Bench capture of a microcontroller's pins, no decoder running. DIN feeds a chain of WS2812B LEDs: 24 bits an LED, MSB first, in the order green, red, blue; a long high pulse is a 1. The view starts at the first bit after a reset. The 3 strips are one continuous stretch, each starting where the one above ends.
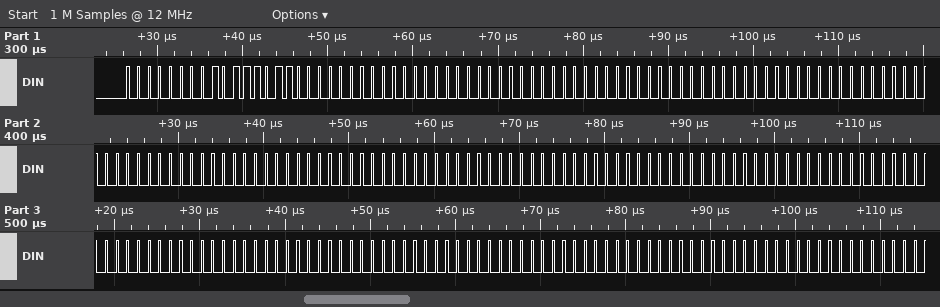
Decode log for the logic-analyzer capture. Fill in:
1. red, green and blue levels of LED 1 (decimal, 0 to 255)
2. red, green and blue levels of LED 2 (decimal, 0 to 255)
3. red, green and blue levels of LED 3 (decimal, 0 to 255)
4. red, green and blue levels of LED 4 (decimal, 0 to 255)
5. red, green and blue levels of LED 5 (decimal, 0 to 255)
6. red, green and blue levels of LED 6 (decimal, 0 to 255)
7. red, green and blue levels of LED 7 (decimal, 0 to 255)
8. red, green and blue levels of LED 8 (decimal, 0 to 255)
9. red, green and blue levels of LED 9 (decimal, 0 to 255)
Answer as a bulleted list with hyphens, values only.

- 187, 0, 0
- 0, 0, 0
- 0, 0, 0
- 0, 0, 0
- 0, 0, 0
- 0, 0, 0
- 0, 0, 0
- 0, 0, 0
- 0, 0, 0
